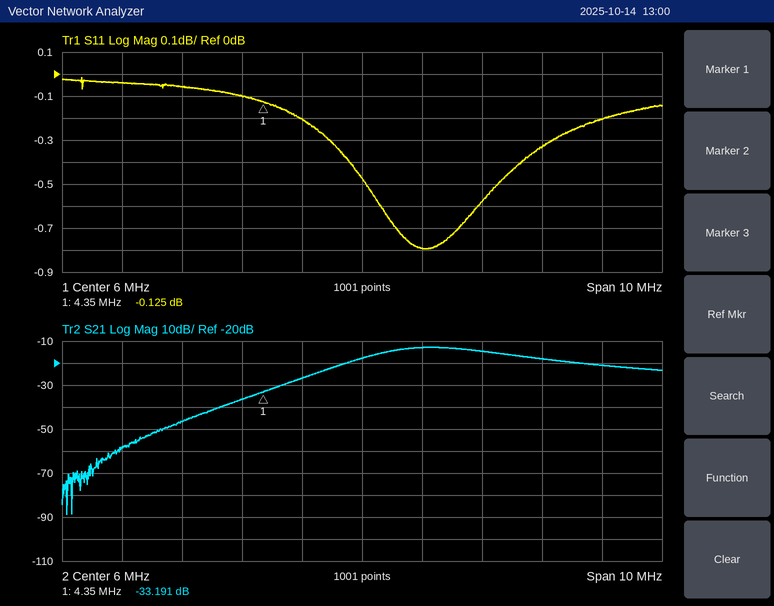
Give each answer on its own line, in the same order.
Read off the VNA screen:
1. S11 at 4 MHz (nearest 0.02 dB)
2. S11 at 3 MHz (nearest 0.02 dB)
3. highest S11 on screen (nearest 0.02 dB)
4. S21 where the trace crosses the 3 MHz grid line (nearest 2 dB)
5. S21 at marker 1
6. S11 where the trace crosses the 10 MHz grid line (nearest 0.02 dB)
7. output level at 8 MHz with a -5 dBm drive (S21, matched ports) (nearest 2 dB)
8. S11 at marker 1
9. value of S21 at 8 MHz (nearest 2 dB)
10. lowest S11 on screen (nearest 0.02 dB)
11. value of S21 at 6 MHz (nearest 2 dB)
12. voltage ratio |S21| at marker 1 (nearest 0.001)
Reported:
-0.10 dB
-0.06 dB
-0.02 dB
-46 dB
-33.191 dB
-0.20 dB
-20 dBm
-0.125 dB
-14 dB
-0.80 dB
-18 dB
0.022
